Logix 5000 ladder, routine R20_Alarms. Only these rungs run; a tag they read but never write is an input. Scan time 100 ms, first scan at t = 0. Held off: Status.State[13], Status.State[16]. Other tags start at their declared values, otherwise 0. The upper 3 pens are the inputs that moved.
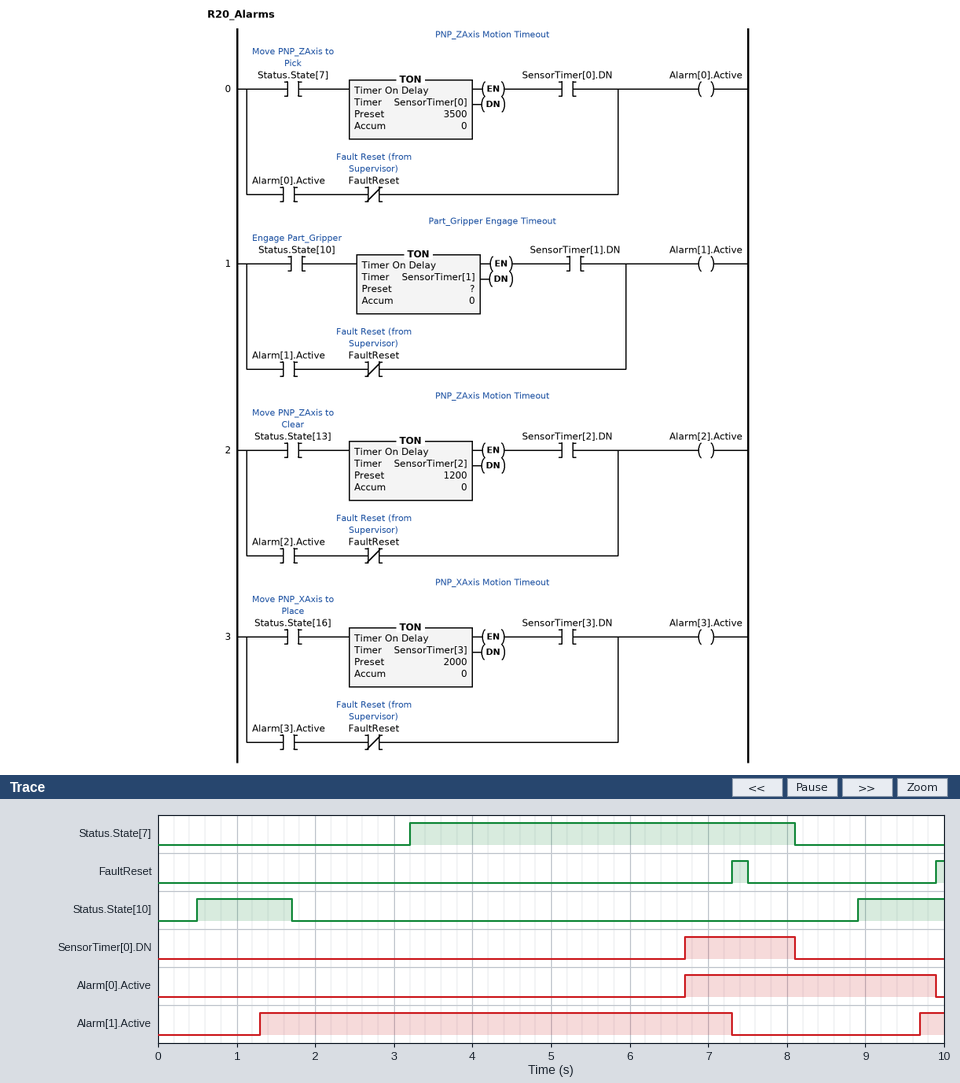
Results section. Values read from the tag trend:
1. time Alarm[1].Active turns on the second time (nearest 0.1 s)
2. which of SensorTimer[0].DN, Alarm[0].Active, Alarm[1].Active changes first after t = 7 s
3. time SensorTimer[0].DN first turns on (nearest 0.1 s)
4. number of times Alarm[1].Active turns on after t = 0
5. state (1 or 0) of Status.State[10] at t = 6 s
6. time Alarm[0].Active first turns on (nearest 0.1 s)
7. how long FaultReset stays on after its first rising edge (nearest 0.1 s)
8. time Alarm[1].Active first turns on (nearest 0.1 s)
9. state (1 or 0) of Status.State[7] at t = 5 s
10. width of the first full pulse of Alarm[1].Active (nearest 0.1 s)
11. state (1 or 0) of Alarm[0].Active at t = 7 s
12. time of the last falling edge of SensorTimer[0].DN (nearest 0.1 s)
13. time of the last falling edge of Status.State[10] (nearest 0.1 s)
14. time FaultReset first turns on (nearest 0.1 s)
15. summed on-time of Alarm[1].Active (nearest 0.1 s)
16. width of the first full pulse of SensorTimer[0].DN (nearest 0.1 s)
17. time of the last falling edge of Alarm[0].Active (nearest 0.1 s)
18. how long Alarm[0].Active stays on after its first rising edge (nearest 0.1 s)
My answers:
9.7 s
Alarm[1].Active
6.7 s
2
0
6.7 s
0.2 s
1.3 s
1
6.0 s
1
8.1 s
1.7 s
7.3 s
6.3 s
1.4 s
9.9 s
3.2 s
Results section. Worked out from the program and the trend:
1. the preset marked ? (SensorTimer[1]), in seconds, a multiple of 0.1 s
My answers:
0.8 s
